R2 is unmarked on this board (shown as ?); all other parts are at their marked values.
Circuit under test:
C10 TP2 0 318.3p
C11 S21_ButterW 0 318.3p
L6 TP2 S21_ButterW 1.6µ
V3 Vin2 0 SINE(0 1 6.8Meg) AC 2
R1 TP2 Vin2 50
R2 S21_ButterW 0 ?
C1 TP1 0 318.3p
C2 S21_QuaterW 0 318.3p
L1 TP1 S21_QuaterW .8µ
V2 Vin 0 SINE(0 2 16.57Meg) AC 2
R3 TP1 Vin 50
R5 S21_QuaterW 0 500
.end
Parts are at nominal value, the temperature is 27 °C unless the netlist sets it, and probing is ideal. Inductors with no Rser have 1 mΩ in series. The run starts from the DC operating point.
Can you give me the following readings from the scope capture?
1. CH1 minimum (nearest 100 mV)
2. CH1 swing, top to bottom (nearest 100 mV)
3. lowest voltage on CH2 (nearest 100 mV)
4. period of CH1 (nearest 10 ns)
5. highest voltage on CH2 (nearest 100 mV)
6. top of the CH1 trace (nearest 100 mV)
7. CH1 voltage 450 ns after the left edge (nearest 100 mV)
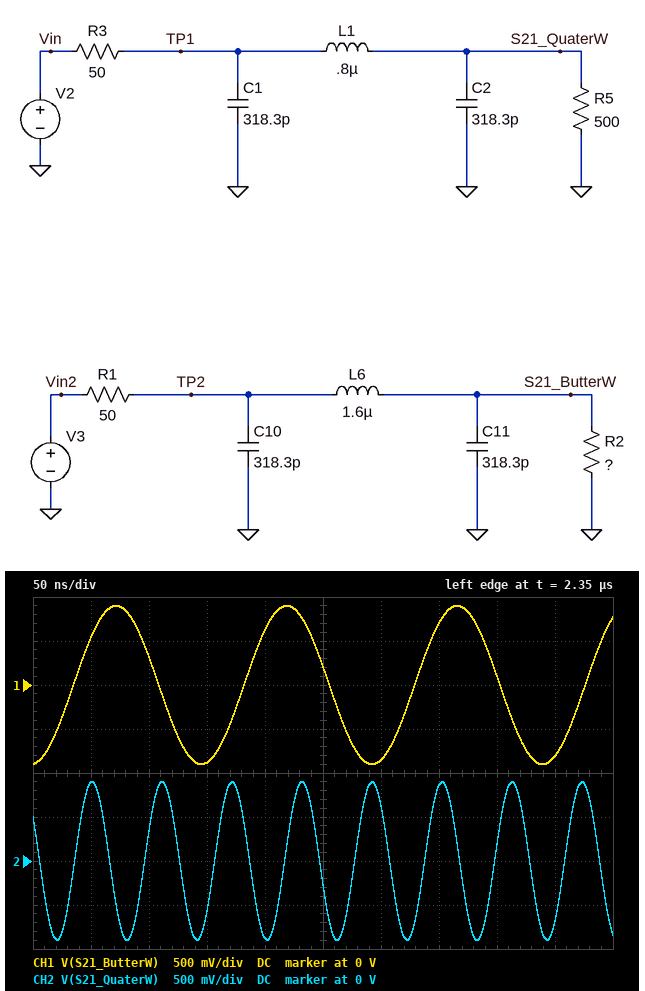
-900 mV
1.8 V
-900 mV
150 ns
900 mV
900 mV
-800 mV
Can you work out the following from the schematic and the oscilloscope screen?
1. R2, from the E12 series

180 Ω
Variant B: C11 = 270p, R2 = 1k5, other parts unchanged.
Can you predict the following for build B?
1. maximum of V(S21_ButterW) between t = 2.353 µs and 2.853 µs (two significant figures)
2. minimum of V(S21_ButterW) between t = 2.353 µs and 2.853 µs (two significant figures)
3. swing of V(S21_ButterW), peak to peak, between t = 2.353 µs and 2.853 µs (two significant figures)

1.3 V
-1.3 V
2.5 V
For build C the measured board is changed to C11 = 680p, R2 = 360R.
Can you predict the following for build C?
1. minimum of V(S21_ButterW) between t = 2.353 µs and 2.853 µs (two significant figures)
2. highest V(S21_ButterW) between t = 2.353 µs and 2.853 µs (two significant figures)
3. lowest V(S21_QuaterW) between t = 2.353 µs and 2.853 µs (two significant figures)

-730 mV
730 mV
-900 mV
